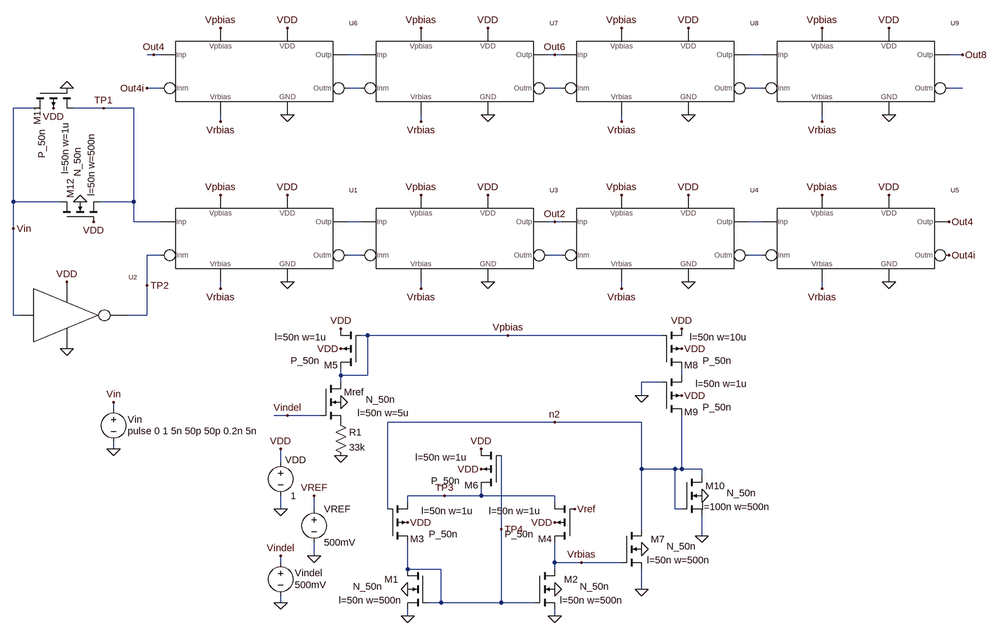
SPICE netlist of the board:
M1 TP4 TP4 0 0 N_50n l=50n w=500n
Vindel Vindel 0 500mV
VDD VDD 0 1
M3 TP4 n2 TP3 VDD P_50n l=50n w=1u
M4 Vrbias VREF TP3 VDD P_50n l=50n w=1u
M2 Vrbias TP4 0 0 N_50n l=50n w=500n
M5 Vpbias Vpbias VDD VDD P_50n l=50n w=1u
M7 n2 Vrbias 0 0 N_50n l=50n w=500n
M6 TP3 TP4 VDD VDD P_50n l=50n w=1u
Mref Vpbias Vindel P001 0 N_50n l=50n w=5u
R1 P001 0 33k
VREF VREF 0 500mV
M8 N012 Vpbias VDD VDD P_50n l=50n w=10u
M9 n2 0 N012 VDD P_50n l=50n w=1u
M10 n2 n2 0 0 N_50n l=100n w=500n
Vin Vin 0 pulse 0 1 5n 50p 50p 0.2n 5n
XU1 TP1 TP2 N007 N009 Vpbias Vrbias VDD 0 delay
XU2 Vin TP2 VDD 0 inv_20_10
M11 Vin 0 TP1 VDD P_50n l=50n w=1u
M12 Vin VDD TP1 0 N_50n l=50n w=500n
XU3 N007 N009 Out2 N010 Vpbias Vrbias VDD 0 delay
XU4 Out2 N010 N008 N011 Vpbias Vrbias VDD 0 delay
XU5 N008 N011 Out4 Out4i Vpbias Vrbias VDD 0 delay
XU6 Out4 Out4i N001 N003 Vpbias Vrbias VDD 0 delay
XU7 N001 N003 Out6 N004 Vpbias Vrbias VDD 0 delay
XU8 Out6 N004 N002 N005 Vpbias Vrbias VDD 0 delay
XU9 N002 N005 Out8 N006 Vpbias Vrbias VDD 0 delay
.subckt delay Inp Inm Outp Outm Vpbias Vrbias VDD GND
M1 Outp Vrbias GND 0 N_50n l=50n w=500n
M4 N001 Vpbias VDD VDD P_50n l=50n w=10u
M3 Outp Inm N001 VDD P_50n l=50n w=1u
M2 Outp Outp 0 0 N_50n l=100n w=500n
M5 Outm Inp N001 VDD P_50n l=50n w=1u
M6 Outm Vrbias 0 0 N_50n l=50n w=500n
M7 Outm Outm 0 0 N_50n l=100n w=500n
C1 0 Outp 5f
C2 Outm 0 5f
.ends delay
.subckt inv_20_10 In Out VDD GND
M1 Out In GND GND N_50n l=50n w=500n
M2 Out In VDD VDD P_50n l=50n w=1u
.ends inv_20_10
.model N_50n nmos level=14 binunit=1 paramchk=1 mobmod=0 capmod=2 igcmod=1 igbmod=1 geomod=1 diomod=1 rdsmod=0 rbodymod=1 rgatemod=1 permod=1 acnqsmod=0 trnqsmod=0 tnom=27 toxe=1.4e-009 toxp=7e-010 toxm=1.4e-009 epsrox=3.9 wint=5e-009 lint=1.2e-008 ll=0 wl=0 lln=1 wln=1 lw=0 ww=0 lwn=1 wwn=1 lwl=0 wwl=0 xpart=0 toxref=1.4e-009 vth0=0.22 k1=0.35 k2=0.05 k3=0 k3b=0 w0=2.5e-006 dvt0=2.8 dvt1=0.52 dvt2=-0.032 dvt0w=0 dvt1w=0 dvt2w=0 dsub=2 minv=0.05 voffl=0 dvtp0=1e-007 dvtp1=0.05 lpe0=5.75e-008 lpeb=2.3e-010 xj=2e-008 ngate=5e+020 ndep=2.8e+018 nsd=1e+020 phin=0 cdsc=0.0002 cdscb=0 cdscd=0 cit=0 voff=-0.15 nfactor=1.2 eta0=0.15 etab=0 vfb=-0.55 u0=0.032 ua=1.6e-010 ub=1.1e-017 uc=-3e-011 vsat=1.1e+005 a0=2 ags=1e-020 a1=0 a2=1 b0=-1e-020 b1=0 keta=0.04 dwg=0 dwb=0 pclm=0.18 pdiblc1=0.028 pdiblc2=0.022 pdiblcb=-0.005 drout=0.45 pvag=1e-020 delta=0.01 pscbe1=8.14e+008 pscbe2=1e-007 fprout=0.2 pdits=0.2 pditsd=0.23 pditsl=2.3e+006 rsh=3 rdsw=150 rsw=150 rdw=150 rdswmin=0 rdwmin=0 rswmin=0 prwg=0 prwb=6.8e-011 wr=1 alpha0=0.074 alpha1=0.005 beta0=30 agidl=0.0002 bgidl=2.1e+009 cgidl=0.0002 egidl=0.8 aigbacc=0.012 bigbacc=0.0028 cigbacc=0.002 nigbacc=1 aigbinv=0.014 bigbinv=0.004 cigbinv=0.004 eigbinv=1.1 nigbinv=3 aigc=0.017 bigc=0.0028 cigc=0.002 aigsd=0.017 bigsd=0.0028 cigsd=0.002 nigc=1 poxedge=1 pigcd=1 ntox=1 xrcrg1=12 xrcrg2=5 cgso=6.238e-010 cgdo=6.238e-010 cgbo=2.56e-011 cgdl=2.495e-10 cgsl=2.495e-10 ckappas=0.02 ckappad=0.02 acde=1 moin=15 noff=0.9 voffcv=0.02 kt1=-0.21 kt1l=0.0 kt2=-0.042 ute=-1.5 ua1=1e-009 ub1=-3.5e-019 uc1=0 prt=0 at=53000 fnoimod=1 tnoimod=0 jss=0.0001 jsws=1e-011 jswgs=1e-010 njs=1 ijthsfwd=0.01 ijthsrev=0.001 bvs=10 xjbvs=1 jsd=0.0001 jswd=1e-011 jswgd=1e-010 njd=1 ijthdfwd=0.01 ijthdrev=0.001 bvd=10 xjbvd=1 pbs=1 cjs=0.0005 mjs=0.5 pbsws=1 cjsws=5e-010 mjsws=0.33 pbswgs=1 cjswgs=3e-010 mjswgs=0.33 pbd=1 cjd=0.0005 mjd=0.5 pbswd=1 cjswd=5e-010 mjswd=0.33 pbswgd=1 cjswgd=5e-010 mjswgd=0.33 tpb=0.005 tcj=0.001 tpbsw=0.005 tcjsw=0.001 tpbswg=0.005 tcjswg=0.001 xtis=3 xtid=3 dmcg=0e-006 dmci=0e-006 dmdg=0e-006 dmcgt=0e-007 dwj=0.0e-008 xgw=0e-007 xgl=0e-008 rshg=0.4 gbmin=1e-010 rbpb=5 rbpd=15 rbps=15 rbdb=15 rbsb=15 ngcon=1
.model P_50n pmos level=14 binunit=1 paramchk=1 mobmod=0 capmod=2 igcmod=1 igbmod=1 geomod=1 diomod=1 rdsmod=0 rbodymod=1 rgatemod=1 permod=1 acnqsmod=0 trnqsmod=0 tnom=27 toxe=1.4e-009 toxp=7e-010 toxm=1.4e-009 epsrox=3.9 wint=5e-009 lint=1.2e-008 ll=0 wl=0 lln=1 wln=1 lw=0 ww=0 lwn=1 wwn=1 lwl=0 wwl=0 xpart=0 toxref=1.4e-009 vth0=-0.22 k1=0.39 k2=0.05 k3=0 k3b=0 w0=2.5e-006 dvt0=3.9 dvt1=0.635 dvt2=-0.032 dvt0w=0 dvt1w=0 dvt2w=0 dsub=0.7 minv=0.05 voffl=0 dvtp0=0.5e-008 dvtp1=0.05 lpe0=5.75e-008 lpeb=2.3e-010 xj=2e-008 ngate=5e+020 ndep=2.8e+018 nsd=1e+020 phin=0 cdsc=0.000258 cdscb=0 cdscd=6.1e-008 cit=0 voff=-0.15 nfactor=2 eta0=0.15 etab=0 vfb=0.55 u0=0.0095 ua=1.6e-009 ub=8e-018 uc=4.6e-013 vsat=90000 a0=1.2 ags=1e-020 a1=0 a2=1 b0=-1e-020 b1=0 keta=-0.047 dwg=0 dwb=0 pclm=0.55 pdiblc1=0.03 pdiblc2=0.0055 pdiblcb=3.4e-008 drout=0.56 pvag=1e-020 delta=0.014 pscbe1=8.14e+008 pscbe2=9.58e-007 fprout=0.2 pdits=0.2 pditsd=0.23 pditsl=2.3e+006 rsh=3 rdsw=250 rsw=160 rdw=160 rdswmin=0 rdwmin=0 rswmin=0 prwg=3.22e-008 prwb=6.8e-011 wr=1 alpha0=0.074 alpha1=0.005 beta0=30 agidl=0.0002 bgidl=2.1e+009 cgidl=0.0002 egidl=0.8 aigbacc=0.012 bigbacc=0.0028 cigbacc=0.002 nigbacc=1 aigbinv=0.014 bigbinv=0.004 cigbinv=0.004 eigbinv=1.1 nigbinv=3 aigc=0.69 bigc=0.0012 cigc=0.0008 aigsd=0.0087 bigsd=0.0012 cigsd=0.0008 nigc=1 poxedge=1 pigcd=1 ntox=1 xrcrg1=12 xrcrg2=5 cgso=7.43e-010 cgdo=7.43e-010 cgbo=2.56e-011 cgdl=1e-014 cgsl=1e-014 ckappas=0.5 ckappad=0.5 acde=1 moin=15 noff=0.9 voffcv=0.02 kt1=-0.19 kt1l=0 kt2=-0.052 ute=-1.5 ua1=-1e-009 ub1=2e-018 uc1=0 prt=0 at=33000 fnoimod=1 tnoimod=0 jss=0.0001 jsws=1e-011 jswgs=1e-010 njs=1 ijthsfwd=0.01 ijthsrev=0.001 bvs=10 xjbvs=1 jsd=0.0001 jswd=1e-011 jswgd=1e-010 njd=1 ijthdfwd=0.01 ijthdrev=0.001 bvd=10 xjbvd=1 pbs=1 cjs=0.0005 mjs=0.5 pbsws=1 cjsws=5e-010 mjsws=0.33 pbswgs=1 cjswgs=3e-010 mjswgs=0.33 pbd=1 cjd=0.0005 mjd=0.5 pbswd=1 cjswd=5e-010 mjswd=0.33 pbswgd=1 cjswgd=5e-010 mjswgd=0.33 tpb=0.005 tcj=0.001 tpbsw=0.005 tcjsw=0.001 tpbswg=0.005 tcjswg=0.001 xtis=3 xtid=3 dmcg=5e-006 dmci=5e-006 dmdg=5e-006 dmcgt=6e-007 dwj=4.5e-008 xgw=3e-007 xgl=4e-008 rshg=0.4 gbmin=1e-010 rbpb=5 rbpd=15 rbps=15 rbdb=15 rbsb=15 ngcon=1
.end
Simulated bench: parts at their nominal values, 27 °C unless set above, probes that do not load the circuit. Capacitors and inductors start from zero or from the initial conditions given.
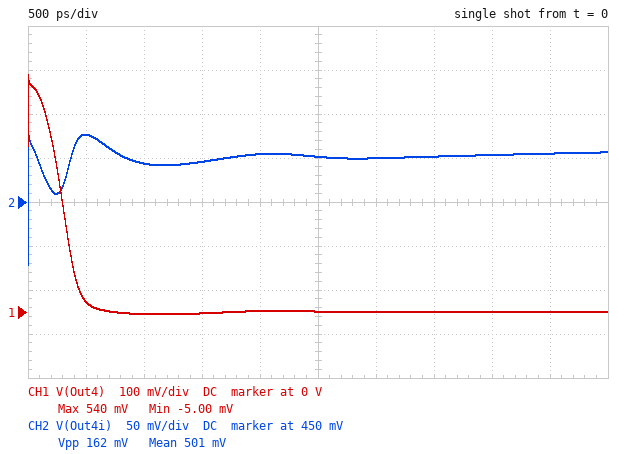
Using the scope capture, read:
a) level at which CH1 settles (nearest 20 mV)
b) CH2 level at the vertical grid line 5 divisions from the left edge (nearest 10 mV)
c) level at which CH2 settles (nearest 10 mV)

0 V
500 mV
510 mV
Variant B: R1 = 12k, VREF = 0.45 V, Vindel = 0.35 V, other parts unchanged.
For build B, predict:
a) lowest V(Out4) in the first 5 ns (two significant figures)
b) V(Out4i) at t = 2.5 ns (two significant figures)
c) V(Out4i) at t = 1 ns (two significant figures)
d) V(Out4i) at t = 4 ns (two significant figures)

-4.6 mV
450 mV
480 mV
460 mV
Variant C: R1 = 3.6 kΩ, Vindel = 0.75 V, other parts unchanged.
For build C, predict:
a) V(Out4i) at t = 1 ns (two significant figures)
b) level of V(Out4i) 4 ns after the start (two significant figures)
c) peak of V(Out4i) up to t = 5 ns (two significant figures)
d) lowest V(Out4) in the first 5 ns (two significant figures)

610 mV
530 mV
660 mV
3.5 mV
